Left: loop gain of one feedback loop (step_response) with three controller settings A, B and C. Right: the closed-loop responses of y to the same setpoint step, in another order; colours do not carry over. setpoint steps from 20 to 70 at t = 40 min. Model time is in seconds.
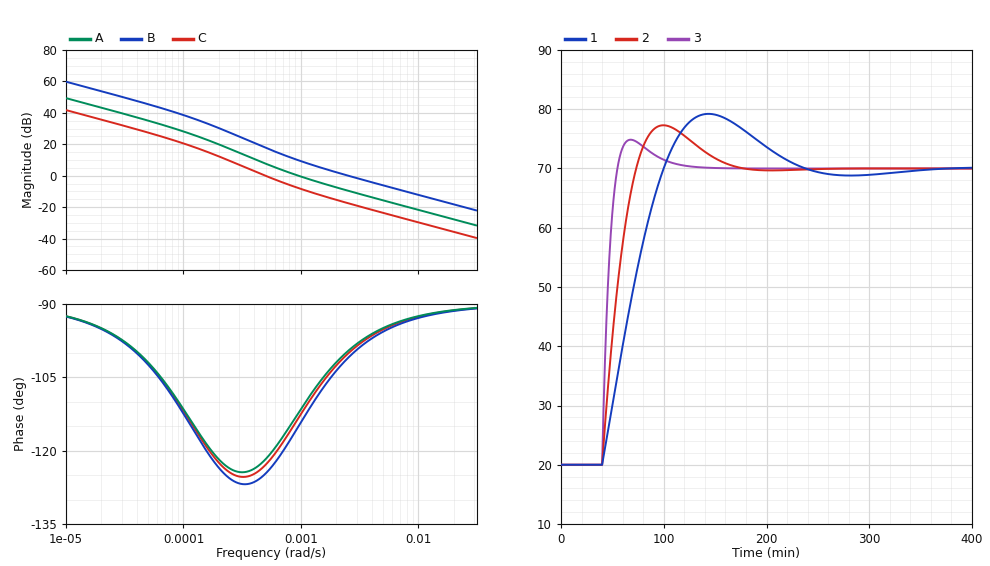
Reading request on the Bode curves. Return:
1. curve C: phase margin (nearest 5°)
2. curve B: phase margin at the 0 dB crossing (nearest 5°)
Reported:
55°
80°
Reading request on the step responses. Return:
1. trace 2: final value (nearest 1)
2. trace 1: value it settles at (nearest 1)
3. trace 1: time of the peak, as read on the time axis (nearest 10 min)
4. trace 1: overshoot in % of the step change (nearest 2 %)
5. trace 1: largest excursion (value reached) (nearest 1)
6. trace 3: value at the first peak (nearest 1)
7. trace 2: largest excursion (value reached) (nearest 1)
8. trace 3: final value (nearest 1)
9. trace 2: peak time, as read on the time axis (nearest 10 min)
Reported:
70
70
140 min
18 %
79
75
77
70
100 min
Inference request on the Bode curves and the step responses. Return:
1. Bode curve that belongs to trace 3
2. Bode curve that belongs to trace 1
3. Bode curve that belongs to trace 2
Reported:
B
C
A
